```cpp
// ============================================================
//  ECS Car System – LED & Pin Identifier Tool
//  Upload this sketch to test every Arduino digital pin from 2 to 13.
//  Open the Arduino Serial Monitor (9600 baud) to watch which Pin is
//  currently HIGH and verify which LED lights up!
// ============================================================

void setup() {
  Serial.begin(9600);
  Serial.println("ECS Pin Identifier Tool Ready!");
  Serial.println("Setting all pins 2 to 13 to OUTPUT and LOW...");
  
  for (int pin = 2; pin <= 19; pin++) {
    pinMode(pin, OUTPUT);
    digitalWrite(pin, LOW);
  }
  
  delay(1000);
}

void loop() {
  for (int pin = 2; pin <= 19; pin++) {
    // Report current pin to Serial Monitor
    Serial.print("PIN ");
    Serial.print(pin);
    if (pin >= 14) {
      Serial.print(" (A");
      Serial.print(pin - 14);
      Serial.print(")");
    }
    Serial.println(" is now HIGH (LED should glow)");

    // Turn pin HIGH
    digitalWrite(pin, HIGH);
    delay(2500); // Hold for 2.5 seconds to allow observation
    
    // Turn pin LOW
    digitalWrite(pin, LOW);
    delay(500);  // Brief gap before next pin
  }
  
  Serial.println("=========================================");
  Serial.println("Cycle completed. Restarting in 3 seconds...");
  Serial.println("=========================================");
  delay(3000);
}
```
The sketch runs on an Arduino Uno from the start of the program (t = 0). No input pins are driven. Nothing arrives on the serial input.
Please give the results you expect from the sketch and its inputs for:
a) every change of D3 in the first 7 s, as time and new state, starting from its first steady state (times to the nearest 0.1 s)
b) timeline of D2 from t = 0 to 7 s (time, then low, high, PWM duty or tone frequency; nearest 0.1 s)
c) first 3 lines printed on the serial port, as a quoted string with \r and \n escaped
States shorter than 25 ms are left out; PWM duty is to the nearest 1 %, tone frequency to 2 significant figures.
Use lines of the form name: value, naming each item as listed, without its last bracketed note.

every change of D3 in the first 7 s, as time and new state, starting from its first steady state: 0 s low; 4 s high; 6.5 s low
timeline of D2 from t = 0 to 7 s: 0 s low; 1 s high; 3.5 s low
first 3 lines printed on the serial port, as a quoted string with \r and \n escaped: "ECS Pin Identifier Tool Ready!\r\nSetting all pins 2 to 13 to OUTPUT and LOW...\r\nPIN 2 is now HIGH (LED should glow)\r\n"
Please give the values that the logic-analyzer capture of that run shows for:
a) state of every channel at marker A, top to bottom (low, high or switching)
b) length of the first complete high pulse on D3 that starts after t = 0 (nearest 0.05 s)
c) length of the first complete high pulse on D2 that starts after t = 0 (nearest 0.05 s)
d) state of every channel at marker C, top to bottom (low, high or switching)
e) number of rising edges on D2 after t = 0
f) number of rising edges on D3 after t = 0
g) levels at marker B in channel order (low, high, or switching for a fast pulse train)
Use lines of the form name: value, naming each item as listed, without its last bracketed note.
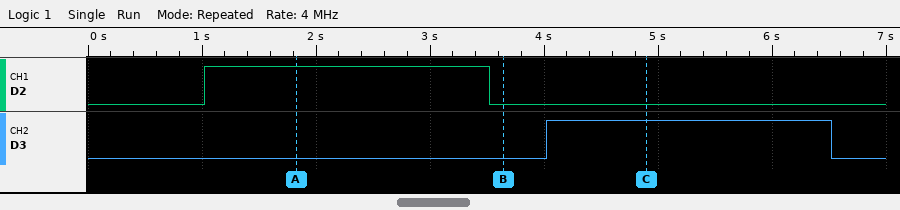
state of every channel at marker A, top to bottom: D2 high, D3 low
length of the first complete high pulse on D3 that starts after t = 0: 2.50 s
length of the first complete high pulse on D2 that starts after t = 0: 2.50 s
state of every channel at marker C, top to bottom: D2 low, D3 high
number of rising edges on D2 after t = 0: 1
number of rising edges on D3 after t = 0: 1
levels at marker B in channel order: D2 low, D3 low
